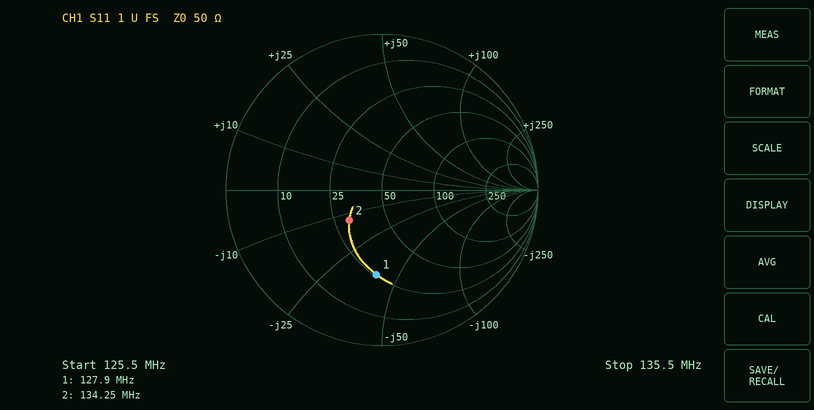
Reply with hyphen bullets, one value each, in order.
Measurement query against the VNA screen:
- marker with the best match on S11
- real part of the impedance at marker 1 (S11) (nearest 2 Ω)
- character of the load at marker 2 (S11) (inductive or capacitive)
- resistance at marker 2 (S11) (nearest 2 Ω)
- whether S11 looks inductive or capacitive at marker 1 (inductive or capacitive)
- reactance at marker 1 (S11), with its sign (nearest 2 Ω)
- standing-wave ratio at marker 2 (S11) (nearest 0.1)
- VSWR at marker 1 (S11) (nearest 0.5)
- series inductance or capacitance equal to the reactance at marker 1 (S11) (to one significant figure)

- marker 2
- 26 Ω
- capacitive
- 30 Ω
- capacitive
- -40 Ω
- 1.8
- 3.5
- 30 pF
